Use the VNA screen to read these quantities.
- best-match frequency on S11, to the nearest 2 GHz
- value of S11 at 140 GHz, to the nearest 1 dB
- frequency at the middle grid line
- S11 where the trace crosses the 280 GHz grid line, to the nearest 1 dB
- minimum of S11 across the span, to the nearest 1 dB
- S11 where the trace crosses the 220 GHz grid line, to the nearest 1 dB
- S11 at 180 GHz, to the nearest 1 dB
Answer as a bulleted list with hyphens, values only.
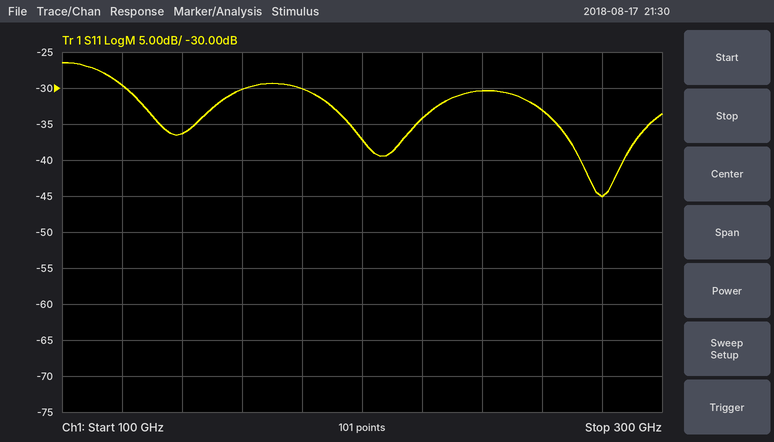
- 280 GHz
- -36 dB
- 200 GHz
- -45 dB
- -45 dB
- -34 dB
- -30 dB
